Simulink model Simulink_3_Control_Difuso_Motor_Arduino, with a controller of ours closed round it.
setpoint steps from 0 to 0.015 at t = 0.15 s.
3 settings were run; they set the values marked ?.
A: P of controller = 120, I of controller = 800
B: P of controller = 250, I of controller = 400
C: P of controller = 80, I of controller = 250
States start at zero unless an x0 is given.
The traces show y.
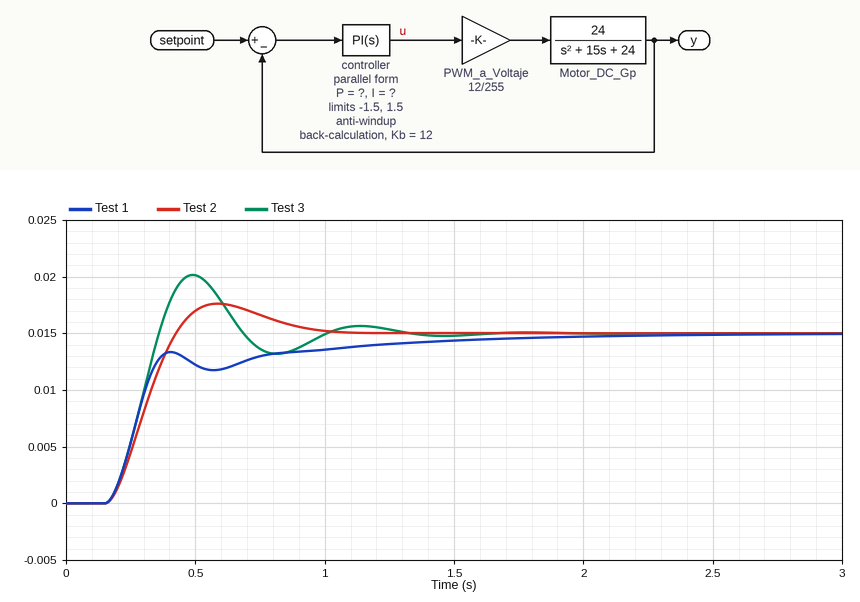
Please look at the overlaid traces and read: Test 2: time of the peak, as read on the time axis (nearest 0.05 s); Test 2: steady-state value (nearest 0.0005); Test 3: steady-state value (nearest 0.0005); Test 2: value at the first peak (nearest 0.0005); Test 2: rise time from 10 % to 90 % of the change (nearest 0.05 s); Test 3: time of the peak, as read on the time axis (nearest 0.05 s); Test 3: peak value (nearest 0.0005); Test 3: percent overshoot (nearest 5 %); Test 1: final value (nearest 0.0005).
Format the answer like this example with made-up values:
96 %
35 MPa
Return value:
0.60 s
0.0150
0.0150
0.0175
0.20 s
0.50 s
0.0200
35 %
0.0150
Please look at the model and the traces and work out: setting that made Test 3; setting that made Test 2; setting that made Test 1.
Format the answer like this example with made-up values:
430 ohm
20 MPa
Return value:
A
C
B
